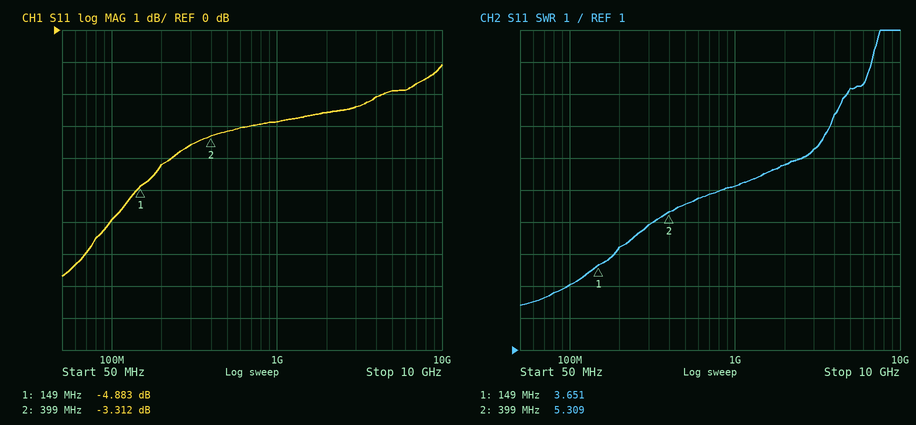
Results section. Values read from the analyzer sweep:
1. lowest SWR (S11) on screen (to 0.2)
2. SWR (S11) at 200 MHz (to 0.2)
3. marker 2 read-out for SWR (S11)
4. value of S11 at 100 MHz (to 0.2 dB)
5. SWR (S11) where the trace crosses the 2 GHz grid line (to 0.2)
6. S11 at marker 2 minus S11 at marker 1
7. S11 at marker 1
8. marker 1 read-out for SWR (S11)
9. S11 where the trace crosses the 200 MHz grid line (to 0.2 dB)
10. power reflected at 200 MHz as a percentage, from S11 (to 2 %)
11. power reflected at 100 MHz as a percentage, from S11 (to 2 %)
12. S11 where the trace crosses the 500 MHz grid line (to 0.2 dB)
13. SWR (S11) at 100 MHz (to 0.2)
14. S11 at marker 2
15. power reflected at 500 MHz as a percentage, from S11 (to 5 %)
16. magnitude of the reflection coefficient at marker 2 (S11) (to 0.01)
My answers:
2.4
4.2
5.309
-6.0 dB
6.8
1.571 dB
-4.883 dB
3.651
-4.2 dB
38 %
26 %
-3.2 dB
3.0
-3.312 dB
50 %
0.68
